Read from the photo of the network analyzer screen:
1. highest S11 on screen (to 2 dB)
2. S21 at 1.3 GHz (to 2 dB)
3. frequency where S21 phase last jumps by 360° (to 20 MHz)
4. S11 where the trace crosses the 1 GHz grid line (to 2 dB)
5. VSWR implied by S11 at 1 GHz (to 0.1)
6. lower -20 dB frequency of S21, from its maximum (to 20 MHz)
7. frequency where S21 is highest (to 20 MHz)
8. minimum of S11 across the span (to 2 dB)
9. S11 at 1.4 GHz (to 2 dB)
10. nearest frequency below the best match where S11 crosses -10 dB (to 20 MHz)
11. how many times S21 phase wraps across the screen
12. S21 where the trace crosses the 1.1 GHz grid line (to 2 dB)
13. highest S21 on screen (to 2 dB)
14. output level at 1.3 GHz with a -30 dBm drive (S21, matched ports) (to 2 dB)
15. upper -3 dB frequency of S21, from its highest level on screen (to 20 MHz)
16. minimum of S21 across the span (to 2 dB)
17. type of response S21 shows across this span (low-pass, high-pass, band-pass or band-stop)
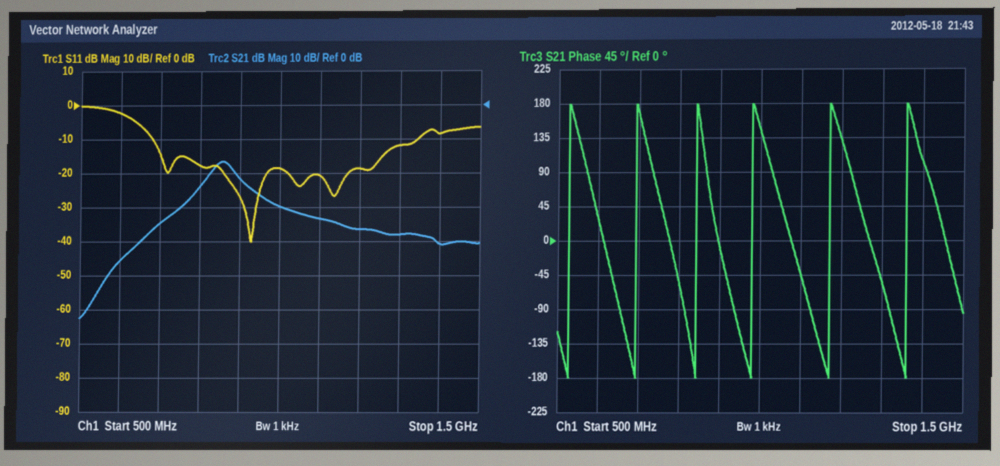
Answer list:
0 dB
-38 dB
1.36 GHz
-18 dB
1.3
680 MHz
860 MHz
-40 dB
-8 dB
680 MHz
6
-34 dB
-16 dB
-68 dBm
880 MHz
-62 dB
band-pass
